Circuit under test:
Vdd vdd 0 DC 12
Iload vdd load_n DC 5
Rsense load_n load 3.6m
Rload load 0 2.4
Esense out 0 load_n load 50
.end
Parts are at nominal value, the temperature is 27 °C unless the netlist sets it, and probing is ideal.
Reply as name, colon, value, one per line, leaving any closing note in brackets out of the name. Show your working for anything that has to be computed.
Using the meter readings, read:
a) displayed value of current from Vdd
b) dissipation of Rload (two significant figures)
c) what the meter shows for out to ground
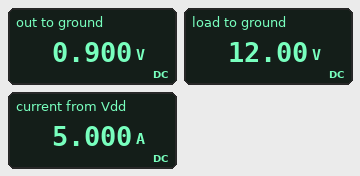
displayed value of current from Vdd: 5.000 A
dissipation of Rload: (12 V)^2 / 2.4 Ω = 60 W
what the meter shows for out to ground: 0.900 V
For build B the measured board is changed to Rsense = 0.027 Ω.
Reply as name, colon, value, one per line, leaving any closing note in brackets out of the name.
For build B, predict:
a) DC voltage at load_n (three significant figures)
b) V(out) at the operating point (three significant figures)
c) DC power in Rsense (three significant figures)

DC voltage at load_n: 12.1 V
V(out) at the operating point: 6.75 V
DC power in Rsense: 675 mW
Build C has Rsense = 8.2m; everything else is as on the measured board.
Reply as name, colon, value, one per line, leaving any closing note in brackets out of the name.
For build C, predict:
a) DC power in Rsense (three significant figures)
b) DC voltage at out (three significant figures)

DC power in Rsense: 205 mW
DC voltage at out: 2.05 V
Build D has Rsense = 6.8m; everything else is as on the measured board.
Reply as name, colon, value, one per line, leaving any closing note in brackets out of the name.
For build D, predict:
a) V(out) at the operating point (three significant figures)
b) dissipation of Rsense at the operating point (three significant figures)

V(out) at the operating point: 1.70 V
dissipation of Rsense at the operating point: 170 mW
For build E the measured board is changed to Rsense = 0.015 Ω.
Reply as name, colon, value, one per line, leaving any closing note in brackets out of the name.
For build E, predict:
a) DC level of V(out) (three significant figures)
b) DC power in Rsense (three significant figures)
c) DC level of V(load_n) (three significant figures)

DC level of V(out): 3.75 V
DC power in Rsense: 375 mW
DC level of V(load_n): 12.1 V
